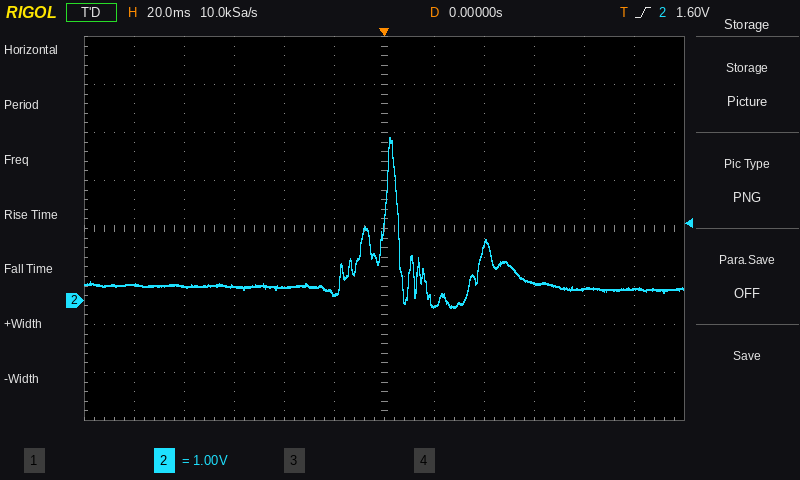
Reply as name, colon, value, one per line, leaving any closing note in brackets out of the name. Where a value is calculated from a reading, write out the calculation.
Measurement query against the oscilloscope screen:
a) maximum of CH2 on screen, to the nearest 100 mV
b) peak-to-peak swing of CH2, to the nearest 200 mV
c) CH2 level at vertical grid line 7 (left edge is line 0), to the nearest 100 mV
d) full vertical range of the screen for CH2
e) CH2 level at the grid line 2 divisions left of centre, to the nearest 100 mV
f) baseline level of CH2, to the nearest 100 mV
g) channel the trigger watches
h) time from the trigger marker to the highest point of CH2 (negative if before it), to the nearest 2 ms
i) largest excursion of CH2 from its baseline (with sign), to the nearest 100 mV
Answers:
maximum of CH2 on screen, to the nearest 100 mV: 3.4 V
peak-to-peak swing of CH2, to the nearest 200 mV: 3.6 V
CH2 level at vertical grid line 7 (left edge is line 0), to the nearest 100 mV: -100 mV
full vertical range of the screen for CH2: 8 V
CH2 level at the grid line 2 divisions left of centre, to the nearest 100 mV: 300 mV
baseline level of CH2, to the nearest 100 mV: 300 mV
channel the trigger watches: CH2
time from the trigger marker to the highest point of CH2 (negative if before it), to the nearest 2 ms: +2 ms
largest excursion of CH2 from its baseline (with sign), to the nearest 100 mV: 3.4 V − (300 mV) = +3.1 V
